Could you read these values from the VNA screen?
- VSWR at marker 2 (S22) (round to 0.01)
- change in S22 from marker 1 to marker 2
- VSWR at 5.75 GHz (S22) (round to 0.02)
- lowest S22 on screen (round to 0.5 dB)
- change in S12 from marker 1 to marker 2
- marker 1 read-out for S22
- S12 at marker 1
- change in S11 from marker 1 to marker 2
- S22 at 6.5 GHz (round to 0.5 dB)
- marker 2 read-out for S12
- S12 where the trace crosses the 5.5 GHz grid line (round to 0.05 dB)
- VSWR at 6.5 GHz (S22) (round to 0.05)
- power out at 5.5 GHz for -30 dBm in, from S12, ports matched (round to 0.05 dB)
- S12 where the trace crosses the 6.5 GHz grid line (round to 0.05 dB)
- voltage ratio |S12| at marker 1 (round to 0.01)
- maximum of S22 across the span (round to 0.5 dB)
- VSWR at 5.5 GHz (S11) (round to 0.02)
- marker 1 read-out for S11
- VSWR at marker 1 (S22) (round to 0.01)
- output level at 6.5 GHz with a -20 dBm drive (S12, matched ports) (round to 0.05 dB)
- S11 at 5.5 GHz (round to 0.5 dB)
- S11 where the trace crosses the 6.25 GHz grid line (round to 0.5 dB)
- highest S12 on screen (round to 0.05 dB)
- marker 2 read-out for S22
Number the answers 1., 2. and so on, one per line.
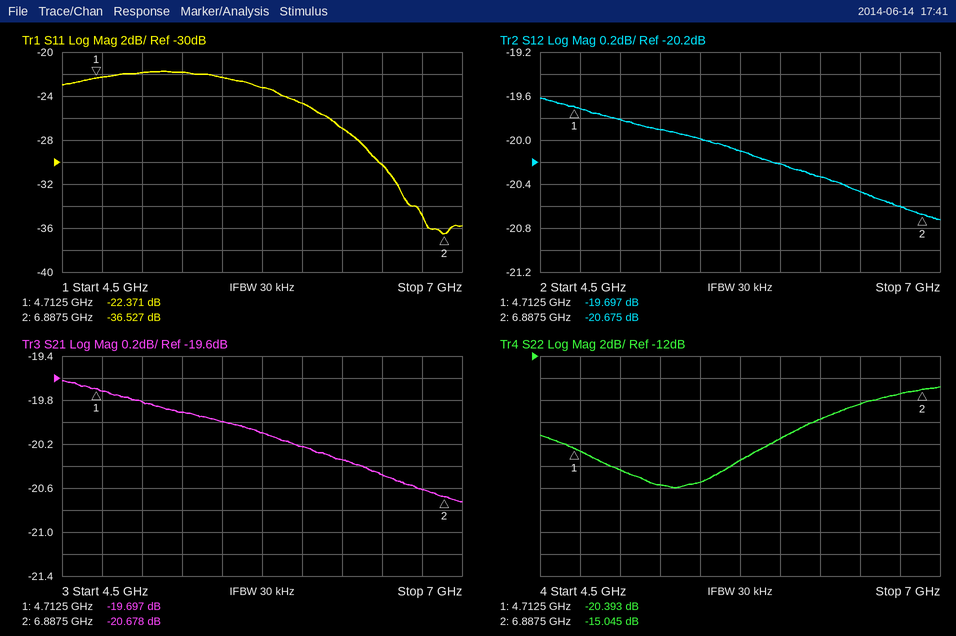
1. 1.43
2. 5.348 dB
3. 1.18
4. -24.0 dB
5. -0.978 dB
6. -20.393 dB
7. -19.697 dB
8. -14.156 dB
9. -16.5 dB
10. -20.675 dB
11. -20.00 dB
12. 1.35
13. -50.00 dBm
14. -20.45 dB
15. 0.10
16. -15.0 dB
17. 1.16
18. -22.371 dB
19. 1.21
20. -40.45 dBm
21. -22.5 dB
22. -27.0 dB
23. -19.60 dB
24. -15.045 dB
